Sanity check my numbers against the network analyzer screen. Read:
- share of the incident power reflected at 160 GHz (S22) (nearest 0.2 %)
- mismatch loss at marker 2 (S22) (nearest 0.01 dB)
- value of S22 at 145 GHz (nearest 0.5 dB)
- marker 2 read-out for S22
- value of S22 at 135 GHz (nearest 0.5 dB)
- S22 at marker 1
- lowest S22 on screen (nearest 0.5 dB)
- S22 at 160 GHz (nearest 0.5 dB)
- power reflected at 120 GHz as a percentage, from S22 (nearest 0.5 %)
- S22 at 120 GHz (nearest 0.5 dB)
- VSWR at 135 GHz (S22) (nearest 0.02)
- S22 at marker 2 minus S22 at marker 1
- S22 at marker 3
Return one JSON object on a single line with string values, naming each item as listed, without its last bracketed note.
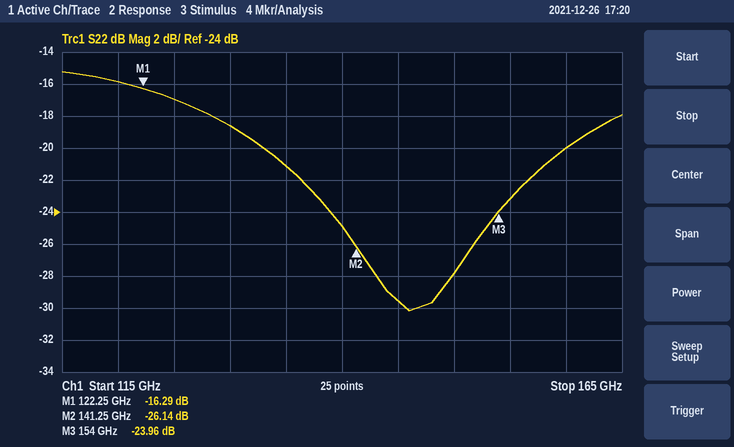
{"share of the incident power reflected at 160 GHz (S22)": "1.0 %", "mismatch loss at marker 2 (S22)": "0.01 dB", "value of S22 at 145 GHz": "-29.5 dB", "marker 2 read-out for S22": "-26.14 dB", "value of S22 at 135 GHz": "-21.0 dB", "S22 at marker 1": "-16.29 dB", "lowest S22 on screen": "-30.0 dB", "S22 at 160 GHz": "-20.0 dB", "power reflected at 120 GHz as a percentage, from S22": "2.5 %", "S22 at 120 GHz": "-16.0 dB", "VSWR at 135 GHz (S22)": "1.20", "S22 at marker 2 minus S22 at marker 1": "-9.85 dB", "S22 at marker 3": "-23.96 dB"}
